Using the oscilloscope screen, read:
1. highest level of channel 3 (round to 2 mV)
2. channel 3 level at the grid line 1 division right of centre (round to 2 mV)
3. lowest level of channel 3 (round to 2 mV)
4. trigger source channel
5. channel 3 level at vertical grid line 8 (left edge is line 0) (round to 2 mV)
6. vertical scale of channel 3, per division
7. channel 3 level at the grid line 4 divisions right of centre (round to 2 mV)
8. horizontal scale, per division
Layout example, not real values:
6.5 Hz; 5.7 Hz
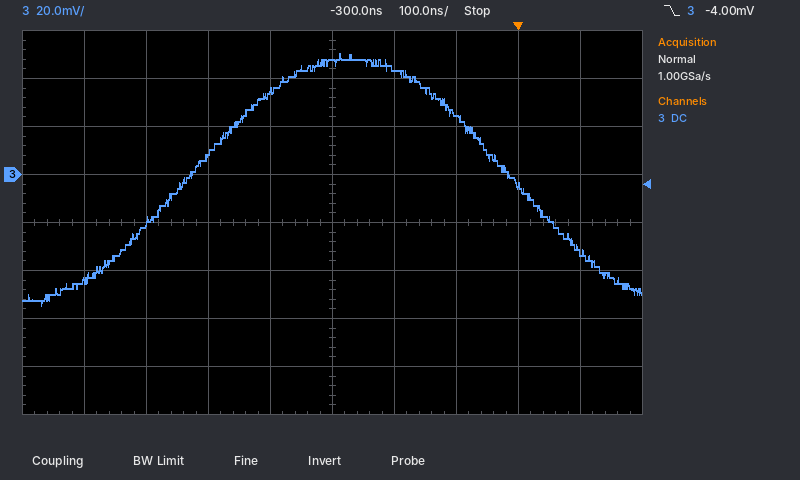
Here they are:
50 mV; 44 mV; -54 mV; channel 3; -4 mV; 20 mV; -32 mV; 100 ns
